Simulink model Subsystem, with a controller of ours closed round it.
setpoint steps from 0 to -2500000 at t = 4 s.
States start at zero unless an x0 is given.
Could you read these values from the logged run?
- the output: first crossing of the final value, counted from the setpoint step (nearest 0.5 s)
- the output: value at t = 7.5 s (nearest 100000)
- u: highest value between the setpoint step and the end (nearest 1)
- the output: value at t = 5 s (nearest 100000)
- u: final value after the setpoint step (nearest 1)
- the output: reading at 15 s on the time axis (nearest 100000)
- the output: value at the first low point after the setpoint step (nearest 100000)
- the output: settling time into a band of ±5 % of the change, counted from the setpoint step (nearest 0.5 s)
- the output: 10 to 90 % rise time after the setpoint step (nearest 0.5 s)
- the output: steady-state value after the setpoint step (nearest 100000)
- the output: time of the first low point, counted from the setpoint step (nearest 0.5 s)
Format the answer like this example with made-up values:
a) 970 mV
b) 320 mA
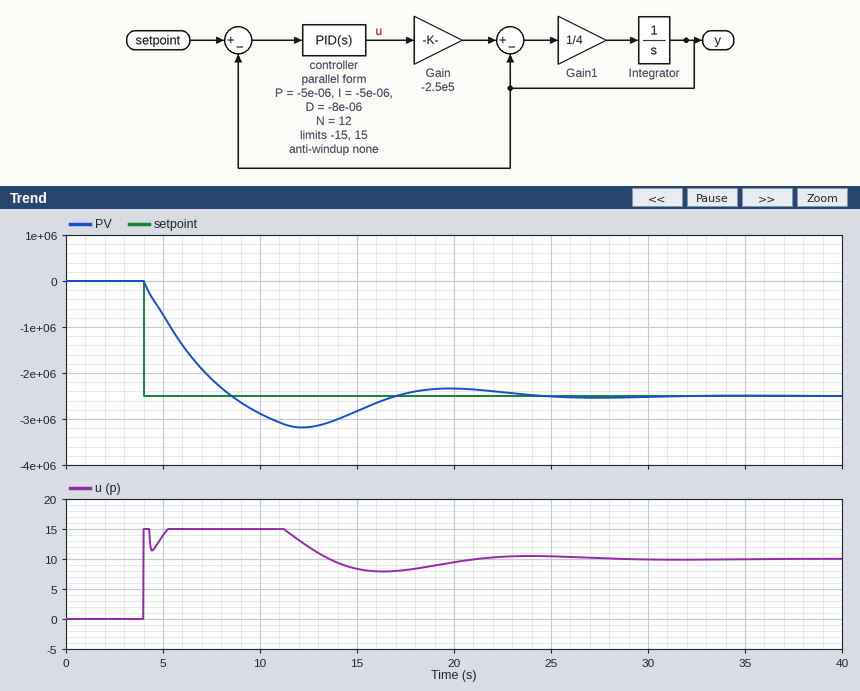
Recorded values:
a) 4.5 s
b) -2100000
c) 15
d) -700000
e) 10
f) -2800000
g) -3200000
h) 17.5 s
i) 3.5 s
j) -2500000
k) 8.0 s
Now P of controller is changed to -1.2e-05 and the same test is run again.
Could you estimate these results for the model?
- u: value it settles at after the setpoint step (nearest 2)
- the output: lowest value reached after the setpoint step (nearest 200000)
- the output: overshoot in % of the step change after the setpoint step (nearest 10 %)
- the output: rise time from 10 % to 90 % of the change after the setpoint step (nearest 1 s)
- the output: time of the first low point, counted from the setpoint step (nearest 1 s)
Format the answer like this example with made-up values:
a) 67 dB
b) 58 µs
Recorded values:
a) 10
b) -3000000
c) 20 %
d) 3 s
e) 7 s
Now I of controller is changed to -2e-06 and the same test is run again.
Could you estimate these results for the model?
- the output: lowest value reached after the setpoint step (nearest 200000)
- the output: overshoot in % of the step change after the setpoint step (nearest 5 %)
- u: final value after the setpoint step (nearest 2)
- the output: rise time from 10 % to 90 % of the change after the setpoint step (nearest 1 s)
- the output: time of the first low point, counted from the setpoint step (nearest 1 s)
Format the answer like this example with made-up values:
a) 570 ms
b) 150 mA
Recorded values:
a) -2800000
b) 10 %
c) 10
d) 5 s
e) 11 s
